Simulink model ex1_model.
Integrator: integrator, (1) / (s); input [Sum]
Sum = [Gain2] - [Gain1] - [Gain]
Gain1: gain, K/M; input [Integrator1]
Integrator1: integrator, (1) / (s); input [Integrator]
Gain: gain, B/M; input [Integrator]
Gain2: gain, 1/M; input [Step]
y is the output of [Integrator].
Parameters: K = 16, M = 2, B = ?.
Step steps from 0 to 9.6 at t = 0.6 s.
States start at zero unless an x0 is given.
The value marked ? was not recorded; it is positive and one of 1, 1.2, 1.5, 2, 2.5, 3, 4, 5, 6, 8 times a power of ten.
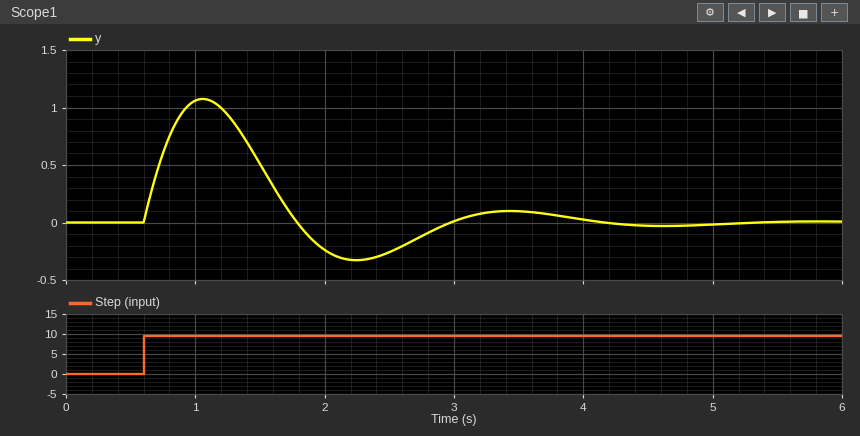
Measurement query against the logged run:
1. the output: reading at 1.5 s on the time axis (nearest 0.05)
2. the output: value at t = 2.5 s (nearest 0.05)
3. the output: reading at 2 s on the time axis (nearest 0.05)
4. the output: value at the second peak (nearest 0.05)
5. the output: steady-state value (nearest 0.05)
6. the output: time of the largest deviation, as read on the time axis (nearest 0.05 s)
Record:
0.50
-0.25
-0.25
0.10
0.00
1.05 s
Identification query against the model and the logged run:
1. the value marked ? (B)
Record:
4
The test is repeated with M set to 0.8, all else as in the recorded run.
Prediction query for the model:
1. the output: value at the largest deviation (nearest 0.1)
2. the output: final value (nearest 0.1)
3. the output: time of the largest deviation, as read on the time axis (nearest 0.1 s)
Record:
1.4
0.0
0.9 s
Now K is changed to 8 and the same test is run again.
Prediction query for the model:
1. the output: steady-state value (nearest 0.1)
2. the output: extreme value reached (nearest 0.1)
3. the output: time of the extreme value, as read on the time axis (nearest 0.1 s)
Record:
0.0
1.3
1.2 s
